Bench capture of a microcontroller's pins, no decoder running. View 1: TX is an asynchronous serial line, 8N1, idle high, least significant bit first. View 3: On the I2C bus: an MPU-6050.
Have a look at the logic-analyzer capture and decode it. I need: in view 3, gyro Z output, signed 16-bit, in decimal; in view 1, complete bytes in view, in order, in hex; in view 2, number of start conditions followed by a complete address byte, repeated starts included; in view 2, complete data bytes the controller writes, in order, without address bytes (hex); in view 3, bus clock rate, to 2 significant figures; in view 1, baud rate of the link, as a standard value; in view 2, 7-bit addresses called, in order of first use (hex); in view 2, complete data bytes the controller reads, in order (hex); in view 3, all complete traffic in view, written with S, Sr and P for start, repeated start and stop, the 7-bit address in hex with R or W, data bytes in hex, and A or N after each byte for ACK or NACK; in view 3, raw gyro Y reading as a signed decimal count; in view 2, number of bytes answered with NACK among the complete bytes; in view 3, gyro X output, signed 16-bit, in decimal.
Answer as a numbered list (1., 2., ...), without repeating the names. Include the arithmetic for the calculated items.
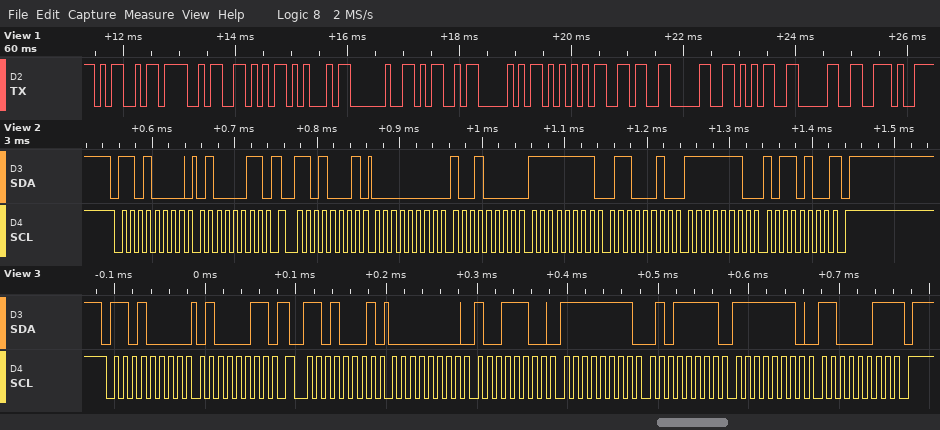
1. 0xFEC3 = -317
2. 0x4D 0x4F 0x56 0x45 0x20 0x4D 0x50 0x55 0x36 0x30 0x35 0x30 0x2E
3. 2
4. 43
5. 100 kHz
6. 9600 baud
7. 0x68
8. 00 90 FF 62 FE B4
9. S 68W A 43 A Sr 68R A 00 A 9C A FF A 5F A FE A C3 N P
10. 0xFF5F = -161
11. 1
12. 0x009C = 156
